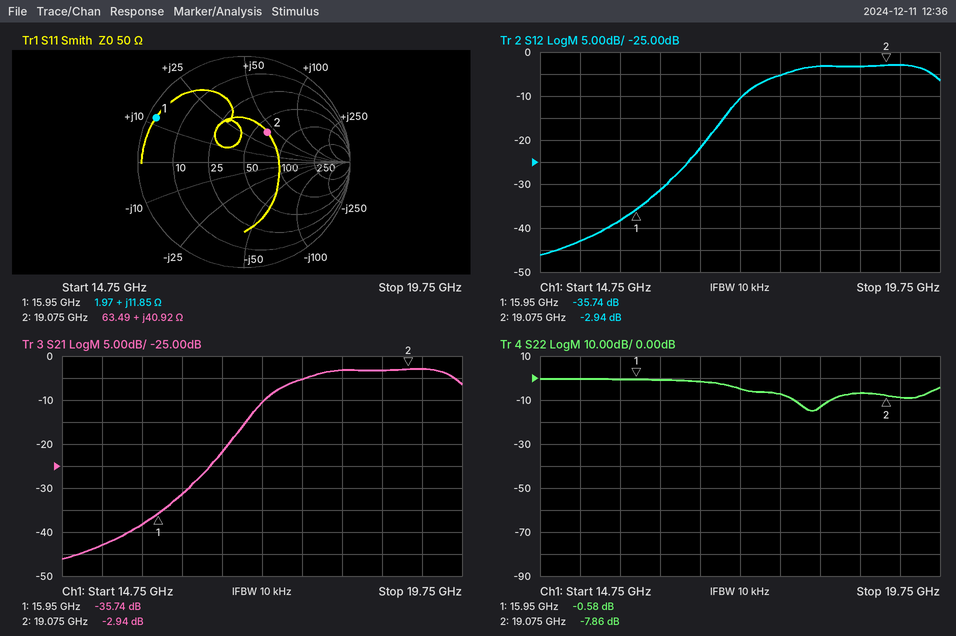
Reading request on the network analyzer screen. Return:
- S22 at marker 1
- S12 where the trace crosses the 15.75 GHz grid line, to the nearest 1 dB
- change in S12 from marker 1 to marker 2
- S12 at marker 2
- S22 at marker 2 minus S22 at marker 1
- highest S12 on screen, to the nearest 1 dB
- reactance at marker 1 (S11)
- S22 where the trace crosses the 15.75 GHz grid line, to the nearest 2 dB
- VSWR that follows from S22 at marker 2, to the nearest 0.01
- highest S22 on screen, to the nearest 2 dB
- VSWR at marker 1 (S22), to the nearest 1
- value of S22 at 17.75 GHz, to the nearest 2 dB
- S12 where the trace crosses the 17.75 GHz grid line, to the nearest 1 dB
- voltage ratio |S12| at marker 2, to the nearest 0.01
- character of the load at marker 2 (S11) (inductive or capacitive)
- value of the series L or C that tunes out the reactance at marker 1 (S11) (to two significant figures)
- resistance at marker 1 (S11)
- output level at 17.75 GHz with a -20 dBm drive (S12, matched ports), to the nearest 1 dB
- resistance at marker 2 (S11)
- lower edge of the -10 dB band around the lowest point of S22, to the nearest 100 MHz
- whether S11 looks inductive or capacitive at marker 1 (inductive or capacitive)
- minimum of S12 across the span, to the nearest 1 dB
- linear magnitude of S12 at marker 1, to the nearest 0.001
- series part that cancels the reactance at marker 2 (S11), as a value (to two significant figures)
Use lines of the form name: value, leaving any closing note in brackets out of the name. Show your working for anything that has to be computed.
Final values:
S22 at marker 1: -0.58 dB
S12 where the trace crosses the 15.75 GHz grid line, to the nearest 1 dB: -38 dB
change in S12 from marker 1 to marker 2: -2.94 − (-35.74) = 32.80 dB
S12 at marker 2: -2.94 dB
S22 at marker 2 minus S22 at marker 1: -7.86 − (-0.58) = -7.28 dB
highest S12 on screen, to the nearest 1 dB: -3 dB
reactance at marker 1: +11.85 Ω
S22 where the trace crosses the 15.75 GHz grid line, to the nearest 2 dB: 0 dB
VSWR that follows from S22 at marker 2, to the nearest 0.01: (1 + 0.4046)/(1 − 0.4046) ≈ 2.36
highest S22 on screen, to the nearest 2 dB: 0 dB
VSWR at marker 1 (S22), to the nearest 1: (1 + 0.9354)/(1 − 0.9354) ≈ 30
value of S22 at 17.75 GHz, to the nearest 2 dB: -8 dB
S12 where the trace crosses the 17.75 GHz grid line, to the nearest 1 dB: -5 dB
voltage ratio |S12| at marker 2, to the nearest 0.01: 10^(-2.94/20) ≈ 0.71
character of the load at marker 2 (S11): inductive
value of the series L or C that tunes out the reactance at marker 1 (S11): C = 1/(2π × 15.95 GHz × 11.85 Ω) ≈ 842 fF, so 840 fF to two significant figures
resistance at marker 1: 1.97 Ω
output level at 17.75 GHz with a -20 dBm drive (S12, matched ports), to the nearest 1 dB: -20 dBm + (-5 dB) = -25 dBm
resistance at marker 2: 63.49 Ω
lower edge of the -10 dB band around the lowest point of S22, to the nearest 100 MHz: 17.9 GHz
whether S11 looks inductive or capacitive at marker 1: inductive
minimum of S12 across the span, to the nearest 1 dB: -46 dB
linear magnitude of S12 at marker 1, to the nearest 0.001: 10^(-35.74/20) ≈ 0.016
series part that cancels the reactance at marker 2 (S11), as a value: C = 1/(2π × 19.075 GHz × 40.92 Ω) ≈ 204 fF, so 200 fF to two significant figures
